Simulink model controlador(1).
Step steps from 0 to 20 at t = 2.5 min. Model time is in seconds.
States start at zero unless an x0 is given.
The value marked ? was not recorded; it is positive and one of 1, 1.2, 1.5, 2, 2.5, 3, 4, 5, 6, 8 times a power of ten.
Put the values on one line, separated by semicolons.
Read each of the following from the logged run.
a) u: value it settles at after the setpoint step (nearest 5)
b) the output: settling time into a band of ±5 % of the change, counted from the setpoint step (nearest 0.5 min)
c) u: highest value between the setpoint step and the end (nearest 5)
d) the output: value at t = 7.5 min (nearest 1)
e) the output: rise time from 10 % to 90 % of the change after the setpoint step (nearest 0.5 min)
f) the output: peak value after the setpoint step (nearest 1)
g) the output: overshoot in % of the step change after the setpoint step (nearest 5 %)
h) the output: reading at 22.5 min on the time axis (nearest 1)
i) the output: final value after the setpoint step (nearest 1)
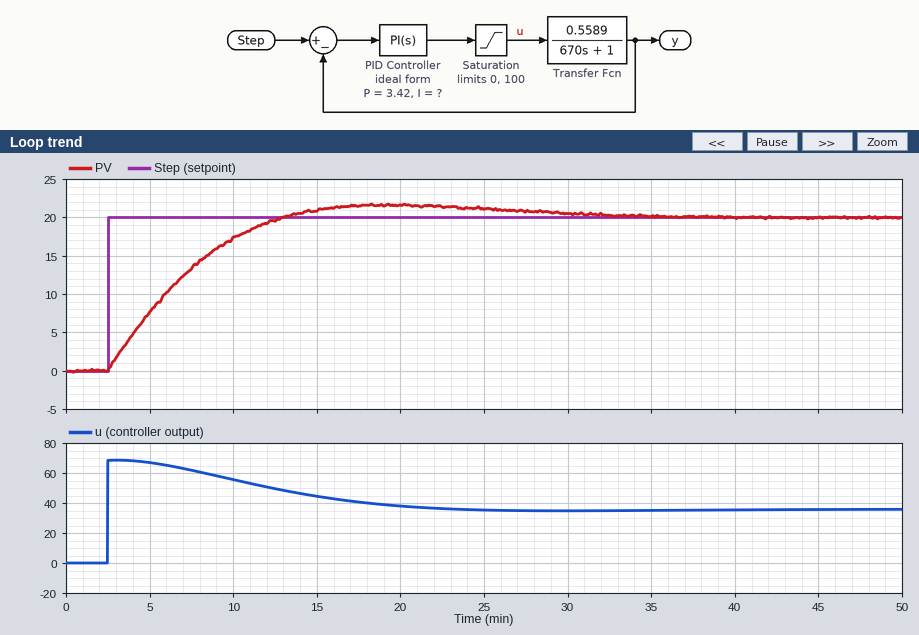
35; 23.5 min; 70; 13; 7.5 min; 22; 10 %; 21; 20
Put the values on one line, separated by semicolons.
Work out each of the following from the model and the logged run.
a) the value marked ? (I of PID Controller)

0.003
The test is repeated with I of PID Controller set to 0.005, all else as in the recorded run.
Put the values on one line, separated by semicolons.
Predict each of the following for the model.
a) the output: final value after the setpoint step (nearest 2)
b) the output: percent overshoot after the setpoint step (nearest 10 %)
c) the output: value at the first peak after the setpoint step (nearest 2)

20; 20 %; 24
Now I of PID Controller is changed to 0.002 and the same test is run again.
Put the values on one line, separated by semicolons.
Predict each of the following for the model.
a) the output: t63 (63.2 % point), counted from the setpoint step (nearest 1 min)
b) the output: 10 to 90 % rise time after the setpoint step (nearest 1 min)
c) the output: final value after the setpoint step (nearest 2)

5 min; 10 min; 20
